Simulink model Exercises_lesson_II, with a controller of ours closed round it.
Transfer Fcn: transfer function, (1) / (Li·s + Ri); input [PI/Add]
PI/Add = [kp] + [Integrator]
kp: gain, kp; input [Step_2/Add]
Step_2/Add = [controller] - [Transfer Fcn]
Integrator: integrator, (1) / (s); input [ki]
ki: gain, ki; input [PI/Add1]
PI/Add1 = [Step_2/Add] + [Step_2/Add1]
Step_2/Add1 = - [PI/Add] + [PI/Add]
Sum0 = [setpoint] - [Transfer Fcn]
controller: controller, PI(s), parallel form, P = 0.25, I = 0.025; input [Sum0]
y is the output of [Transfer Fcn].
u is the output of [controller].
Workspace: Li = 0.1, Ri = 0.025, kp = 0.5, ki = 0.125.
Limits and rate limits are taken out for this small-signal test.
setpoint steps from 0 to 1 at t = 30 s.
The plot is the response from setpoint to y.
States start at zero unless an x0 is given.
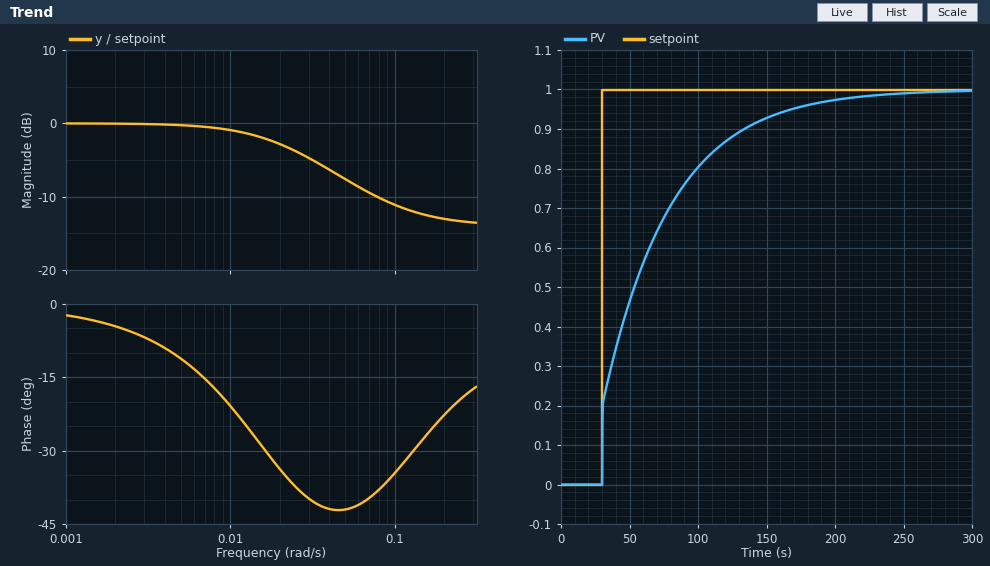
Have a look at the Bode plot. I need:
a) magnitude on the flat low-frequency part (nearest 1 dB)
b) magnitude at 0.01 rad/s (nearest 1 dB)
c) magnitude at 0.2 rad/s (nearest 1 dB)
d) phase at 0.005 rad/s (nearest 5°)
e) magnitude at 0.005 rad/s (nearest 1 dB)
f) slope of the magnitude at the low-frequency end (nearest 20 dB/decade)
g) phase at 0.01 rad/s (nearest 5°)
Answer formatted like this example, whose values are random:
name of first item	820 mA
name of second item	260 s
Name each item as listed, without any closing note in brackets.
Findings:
magnitude on the flat low-frequency part	0 dB
magnitude at 0.01 rad/s	-1 dB
magnitude at 0.2 rad/s	-13 dB
phase at 0.005 rad/s	-10°
magnitude at 0.005 rad/s	0 dB
slope of the magnitude at the low-frequency end	0 dB/decade
phase at 0.01 rad/s	-20°
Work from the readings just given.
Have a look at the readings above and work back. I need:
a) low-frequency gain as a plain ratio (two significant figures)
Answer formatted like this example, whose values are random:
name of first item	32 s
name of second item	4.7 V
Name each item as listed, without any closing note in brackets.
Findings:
low-frequency gain as a plain ratio	1.0
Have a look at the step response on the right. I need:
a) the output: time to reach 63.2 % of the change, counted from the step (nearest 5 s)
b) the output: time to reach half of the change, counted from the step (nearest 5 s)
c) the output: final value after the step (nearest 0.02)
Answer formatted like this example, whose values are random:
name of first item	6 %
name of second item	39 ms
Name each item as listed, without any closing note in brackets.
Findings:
the output: time to reach 63.2 % of the change, counted from the step	40 s
the output: time to reach half of the change, counted from the step	25 s
the output: final value after the step	1.00
